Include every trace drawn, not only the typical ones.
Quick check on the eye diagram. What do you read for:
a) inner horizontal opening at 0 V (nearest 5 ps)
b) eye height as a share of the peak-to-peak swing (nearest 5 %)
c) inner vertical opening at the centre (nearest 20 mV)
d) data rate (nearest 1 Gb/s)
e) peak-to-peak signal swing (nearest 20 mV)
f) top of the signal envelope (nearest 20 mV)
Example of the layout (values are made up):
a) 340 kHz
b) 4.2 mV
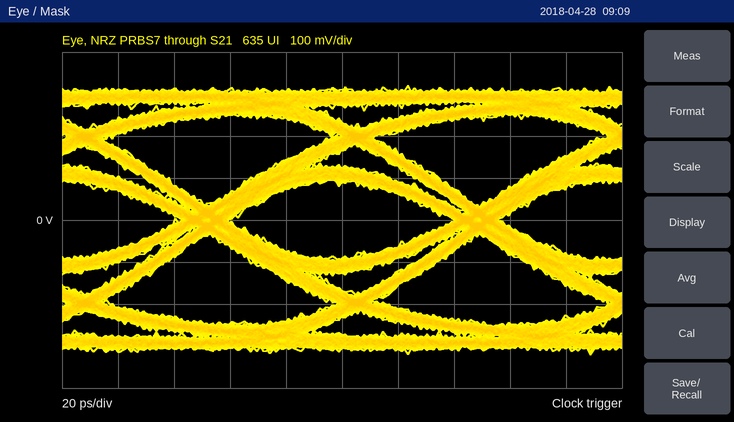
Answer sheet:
a) 80 ps
b) 30 %
c) 180 mV
d) 10 Gb/s
e) 640 mV
f) 320 mV
